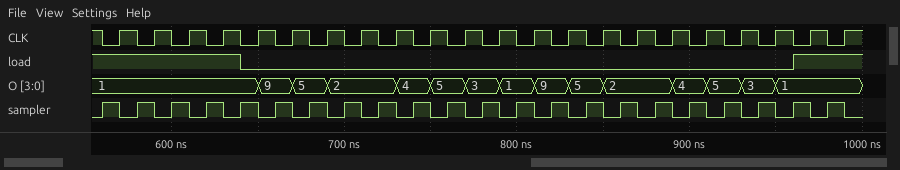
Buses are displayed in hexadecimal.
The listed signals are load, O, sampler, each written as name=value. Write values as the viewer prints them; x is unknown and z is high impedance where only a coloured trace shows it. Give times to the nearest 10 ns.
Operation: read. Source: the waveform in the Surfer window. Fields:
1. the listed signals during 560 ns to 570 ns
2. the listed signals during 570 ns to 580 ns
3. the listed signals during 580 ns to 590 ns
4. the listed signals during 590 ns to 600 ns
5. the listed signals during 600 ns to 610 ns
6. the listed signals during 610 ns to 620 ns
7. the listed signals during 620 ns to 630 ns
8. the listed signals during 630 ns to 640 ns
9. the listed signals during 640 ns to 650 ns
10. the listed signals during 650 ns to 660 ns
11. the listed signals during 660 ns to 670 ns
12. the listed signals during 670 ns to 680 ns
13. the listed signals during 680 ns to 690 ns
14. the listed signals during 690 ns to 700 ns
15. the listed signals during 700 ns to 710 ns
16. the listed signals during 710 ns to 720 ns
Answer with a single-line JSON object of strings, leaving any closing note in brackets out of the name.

{"the listed signals during 560 ns to 570 ns": "load=1, O=1, sampler=1", "the listed signals during 570 ns to 580 ns": "load=1, O=1, sampler=0", "the listed signals during 580 ns to 590 ns": "load=1, O=1, sampler=1", "the listed signals during 590 ns to 600 ns": "load=1, O=1, sampler=0", "the listed signals during 600 ns to 610 ns": "load=1, O=1, sampler=1", "the listed signals during 610 ns to 620 ns": "load=1, O=1, sampler=0", "the listed signals during 620 ns to 630 ns": "load=1, O=1, sampler=1", "the listed signals during 630 ns to 640 ns": "load=1, O=1, sampler=0", "the listed signals during 640 ns to 650 ns": "load=0, O=1, sampler=1", "the listed signals during 650 ns to 660 ns": "load=0, O=9, sampler=0", "the listed signals during 660 ns to 670 ns": "load=0, O=9, sampler=1", "the listed signals during 670 ns to 680 ns": "load=0, O=5, sampler=0", "the listed signals during 680 ns to 690 ns": "load=0, O=5, sampler=1", "the listed signals during 690 ns to 700 ns": "load=0, O=2, sampler=0", "the listed signals during 700 ns to 710 ns": "load=0, O=2, sampler=1", "the listed signals during 710 ns to 720 ns": "load=0, O=2, sampler=0"}
